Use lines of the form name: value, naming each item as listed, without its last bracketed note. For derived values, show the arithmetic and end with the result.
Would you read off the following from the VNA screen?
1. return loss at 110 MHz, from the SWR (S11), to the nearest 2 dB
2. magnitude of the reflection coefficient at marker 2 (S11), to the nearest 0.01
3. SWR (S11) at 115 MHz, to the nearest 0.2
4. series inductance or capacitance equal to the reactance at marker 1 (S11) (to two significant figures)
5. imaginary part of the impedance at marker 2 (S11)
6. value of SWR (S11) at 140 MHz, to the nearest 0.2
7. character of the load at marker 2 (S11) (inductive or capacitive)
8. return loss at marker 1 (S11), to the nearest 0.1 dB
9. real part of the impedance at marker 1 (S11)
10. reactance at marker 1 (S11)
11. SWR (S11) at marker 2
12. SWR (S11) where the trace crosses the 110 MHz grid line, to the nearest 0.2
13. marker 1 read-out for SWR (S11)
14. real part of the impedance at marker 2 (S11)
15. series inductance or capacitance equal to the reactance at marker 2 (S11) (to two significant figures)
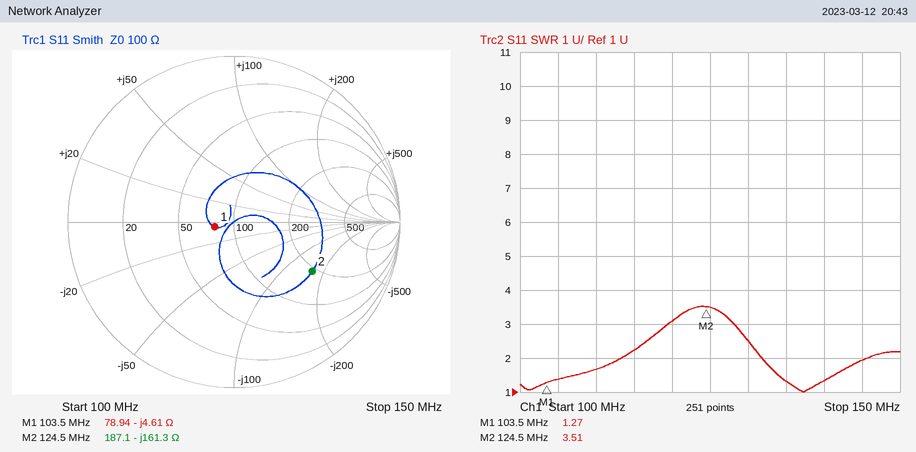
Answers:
return loss at 110 MHz, from the SWR (S11), to the nearest 2 dB: −20 log10((1.6 − 1)/(1.6 + 1)) ≈ 12.7 dB, so 12 dB to the nearest 2 dB
magnitude of the reflection coefficient at marker 2 (S11), to the nearest 0.01: 0.56
SWR (S11) at 115 MHz, to the nearest 0.2: 2.2
series inductance or capacitance equal to the reactance at marker 1 (S11): C = 1/(2π × 103.5 MHz × 4.61 Ω) ≈ 334 pF, so 330 pF to two significant figures
imaginary part of the impedance at marker 2: -161.3 Ω
value of SWR (S11) at 140 MHz, to the nearest 0.2: 1.4
character of the load at marker 2 (S11): capacitive
return loss at marker 1 (S11), to the nearest 0.1 dB: 18.4 dB
real part of the impedance at marker 1: 78.94 Ω
reactance at marker 1: -4.61 Ω
SWR (S11) at marker 2: 3.51
SWR (S11) where the trace crosses the 110 MHz grid line, to the nearest 0.2: 1.6
marker 1 read-out for SWR: 1.27
real part of the impedance at marker 2: 187.1 Ω
series inductance or capacitance equal to the reactance at marker 2 (S11): C = 1/(2π × 124.5 MHz × 161.3 Ω) ≈ 7.9 pF
